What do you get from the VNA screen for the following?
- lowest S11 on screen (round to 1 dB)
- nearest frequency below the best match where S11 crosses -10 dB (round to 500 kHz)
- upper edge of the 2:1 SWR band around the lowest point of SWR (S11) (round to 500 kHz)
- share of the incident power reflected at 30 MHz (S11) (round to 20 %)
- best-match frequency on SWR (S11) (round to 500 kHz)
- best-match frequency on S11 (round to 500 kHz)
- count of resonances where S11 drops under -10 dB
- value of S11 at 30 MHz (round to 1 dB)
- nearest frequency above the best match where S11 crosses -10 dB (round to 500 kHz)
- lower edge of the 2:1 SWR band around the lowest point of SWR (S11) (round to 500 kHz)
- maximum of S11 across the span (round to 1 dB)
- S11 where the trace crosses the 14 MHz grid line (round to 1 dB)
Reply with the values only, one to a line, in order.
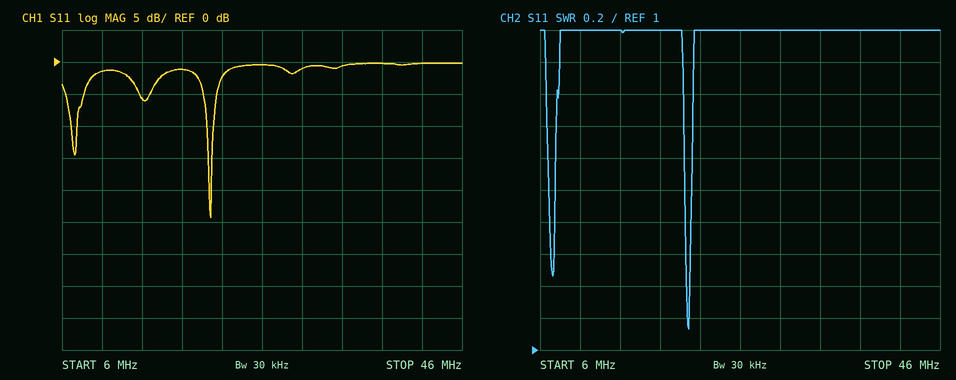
-24 dB
20.5 MHz
21.0 MHz
80 %
21.0 MHz
21.0 MHz
2
-1 dB
21.0 MHz
20.5 MHz
0 dB
-6 dB
